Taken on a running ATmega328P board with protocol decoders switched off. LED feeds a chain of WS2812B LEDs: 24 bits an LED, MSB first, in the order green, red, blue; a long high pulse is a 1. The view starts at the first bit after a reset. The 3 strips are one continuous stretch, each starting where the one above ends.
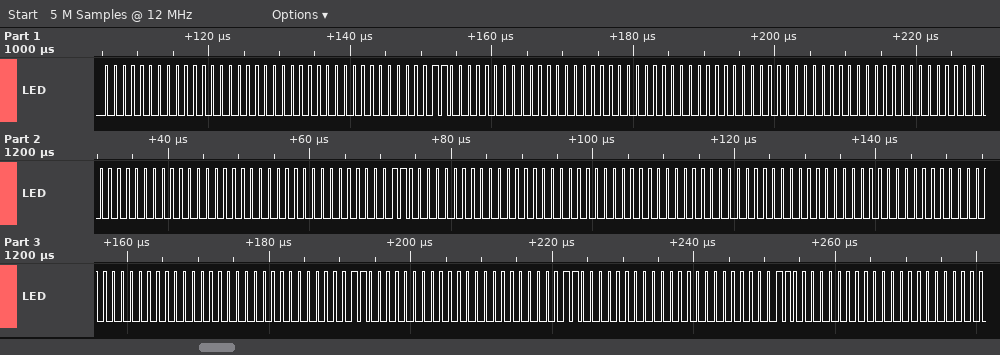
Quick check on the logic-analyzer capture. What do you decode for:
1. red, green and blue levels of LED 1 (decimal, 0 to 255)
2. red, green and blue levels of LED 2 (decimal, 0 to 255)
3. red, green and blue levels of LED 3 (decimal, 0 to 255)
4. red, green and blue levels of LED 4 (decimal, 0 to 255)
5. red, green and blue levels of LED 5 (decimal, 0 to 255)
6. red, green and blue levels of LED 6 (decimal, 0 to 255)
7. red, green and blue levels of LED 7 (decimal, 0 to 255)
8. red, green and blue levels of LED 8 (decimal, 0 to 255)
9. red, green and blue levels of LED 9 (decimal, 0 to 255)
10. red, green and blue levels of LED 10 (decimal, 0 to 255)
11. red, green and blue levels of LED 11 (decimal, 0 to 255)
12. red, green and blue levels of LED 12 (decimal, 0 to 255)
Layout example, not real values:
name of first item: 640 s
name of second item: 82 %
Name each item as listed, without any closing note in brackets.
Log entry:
red, green and blue levels of LED 1: 0, 0, 0
red, green and blue levels of LED 2: 6, 0, 0
red, green and blue levels of LED 3: 0, 0, 0
red, green and blue levels of LED 4: 0, 0, 0
red, green and blue levels of LED 5: 0, 0, 0
red, green and blue levels of LED 6: 6, 0, 0
red, green and blue levels of LED 7: 0, 0, 0
red, green and blue levels of LED 8: 0, 0, 0
red, green and blue levels of LED 9: 0, 0, 0
red, green and blue levels of LED 10: 6, 0, 0
red, green and blue levels of LED 11: 6, 0, 0
red, green and blue levels of LED 12: 6, 0, 0
